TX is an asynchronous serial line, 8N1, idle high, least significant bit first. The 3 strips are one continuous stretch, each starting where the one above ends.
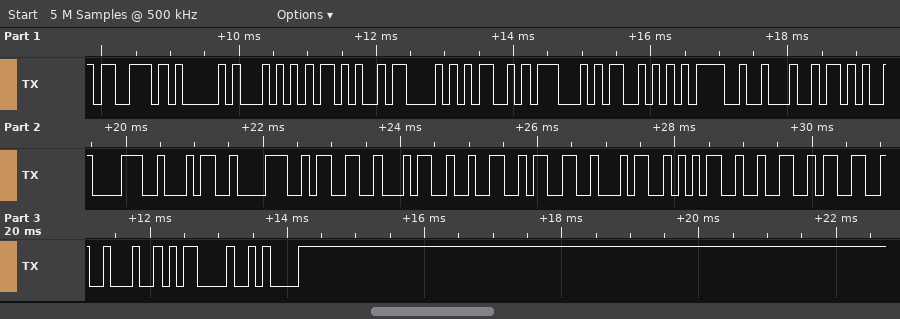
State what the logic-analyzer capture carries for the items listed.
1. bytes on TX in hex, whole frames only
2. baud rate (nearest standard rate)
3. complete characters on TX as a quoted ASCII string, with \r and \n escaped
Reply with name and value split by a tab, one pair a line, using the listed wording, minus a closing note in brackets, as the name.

bytes on TX in hex, whole frames only	73 41 54 2B 43 4D 47 53 3D 22 2B 38 34 38 33 34 32 33 34 35 32 33 22 0D 0A
baud rate	9600 baud
complete characters on TX as a quoted ASCII string, with \r and \n escaped	"sAT+CMGS=\"+84834234523\"\r\n"
